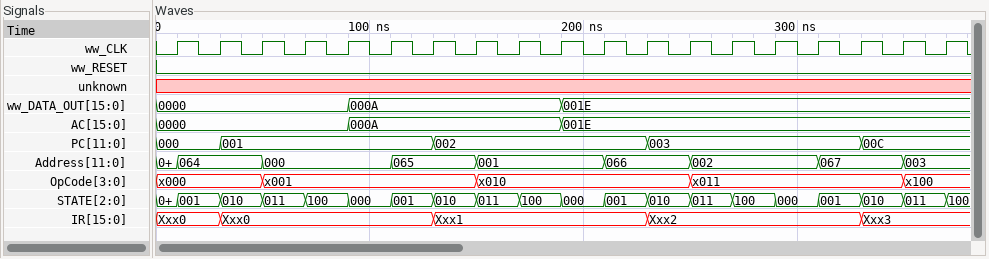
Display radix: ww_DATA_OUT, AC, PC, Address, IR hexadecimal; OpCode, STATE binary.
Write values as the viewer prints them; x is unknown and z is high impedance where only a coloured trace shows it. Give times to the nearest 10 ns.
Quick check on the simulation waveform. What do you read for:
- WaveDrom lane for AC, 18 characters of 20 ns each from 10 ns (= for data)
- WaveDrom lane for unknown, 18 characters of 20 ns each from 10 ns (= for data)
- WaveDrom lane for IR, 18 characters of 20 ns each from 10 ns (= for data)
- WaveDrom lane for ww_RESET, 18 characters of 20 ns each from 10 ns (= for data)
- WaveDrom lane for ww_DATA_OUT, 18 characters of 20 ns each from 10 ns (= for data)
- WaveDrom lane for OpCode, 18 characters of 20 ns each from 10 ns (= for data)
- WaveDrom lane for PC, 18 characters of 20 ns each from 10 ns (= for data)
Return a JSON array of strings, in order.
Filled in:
["{name: 'AC', wave: '=...=....=........', data: '0000 000A 001E'}", "{name: 'unknown', wave: 'x.................'}", "{name: 'IR', wave: '==....=....=....=.', data: 'Xxx0 Xxx0 Xxx1 Xxx2 Xxx3'}", "{name: 'ww_RESET', wave: '0.................'}", "{name: 'ww_DATA_OUT', wave: '=...=....=........', data: '0000 000A 001E'}", "{name: 'OpCode', wave: '=.=....=....=....=', data: 'x000 x001 x010 x011 x100'}", "{name: 'PC', wave: '==....=....=....=.', data: '000 001 002 003 00C'}"]
